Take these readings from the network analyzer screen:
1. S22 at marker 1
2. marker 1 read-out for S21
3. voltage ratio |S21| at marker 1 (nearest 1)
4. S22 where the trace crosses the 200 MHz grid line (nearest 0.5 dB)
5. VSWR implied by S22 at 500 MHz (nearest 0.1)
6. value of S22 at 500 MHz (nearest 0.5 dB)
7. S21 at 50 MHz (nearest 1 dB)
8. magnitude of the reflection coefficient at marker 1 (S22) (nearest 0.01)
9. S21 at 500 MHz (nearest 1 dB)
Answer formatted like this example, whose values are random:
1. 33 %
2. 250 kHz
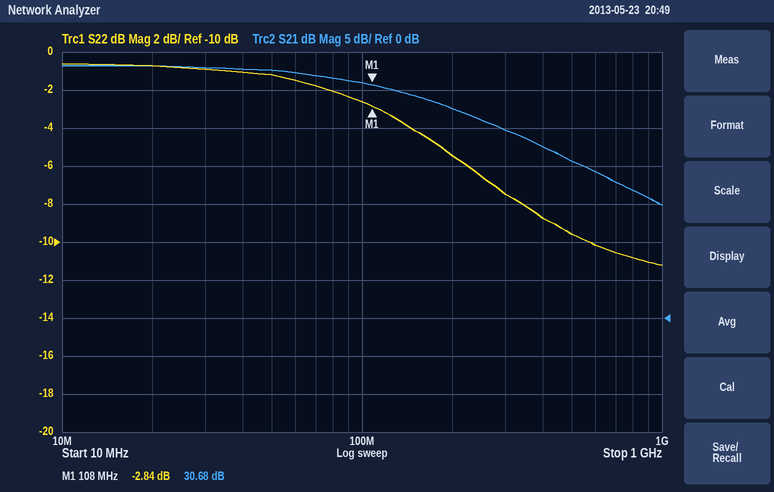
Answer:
1. -2.84 dB
2. 30.68 dB
3. 34
4. -5.5 dB
5. 2.0
6. -9.5 dB
7. 33 dB
8. 0.72
9. 21 dB
